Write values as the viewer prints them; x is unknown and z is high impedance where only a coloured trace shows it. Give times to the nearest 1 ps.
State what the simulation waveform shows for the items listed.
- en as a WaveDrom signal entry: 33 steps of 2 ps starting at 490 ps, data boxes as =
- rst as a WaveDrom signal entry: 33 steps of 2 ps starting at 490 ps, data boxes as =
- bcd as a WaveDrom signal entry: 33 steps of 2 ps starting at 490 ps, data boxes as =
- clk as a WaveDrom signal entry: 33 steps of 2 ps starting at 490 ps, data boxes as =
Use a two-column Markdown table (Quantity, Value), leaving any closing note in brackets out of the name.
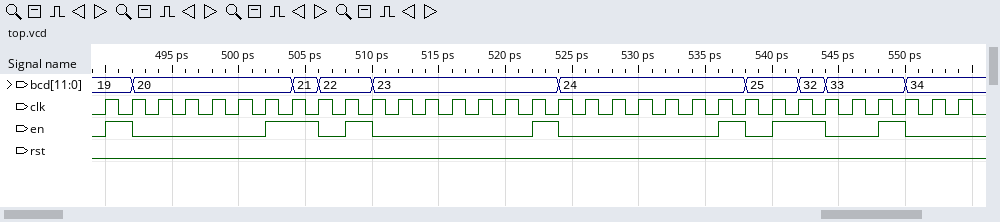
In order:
| Quantity | Value |
|---|---|
| en as a WaveDrom signal entry: 33 steps of 2 ps starting at 490 ps, data boxes as = | {name: 'en', wave: '10....1.010.....10.....101.0.10..'} |
| rst as a WaveDrom signal entry: 33 steps of 2 ps starting at 490 ps, data boxes as = | {name: 'rst', wave: '0................................'} |
| bcd as a WaveDrom signal entry: 33 steps of 2 ps starting at 490 ps, data boxes as = | {name: 'bcd', wave: '==.....==.=......=......=.==..=..', data: '19 20 21 22 23 24 25 32 33 34'} |
| clk as a WaveDrom signal entry: 33 steps of 2 ps starting at 490 ps, data boxes as = | {name: 'clk', wave: 'p................................'} |
